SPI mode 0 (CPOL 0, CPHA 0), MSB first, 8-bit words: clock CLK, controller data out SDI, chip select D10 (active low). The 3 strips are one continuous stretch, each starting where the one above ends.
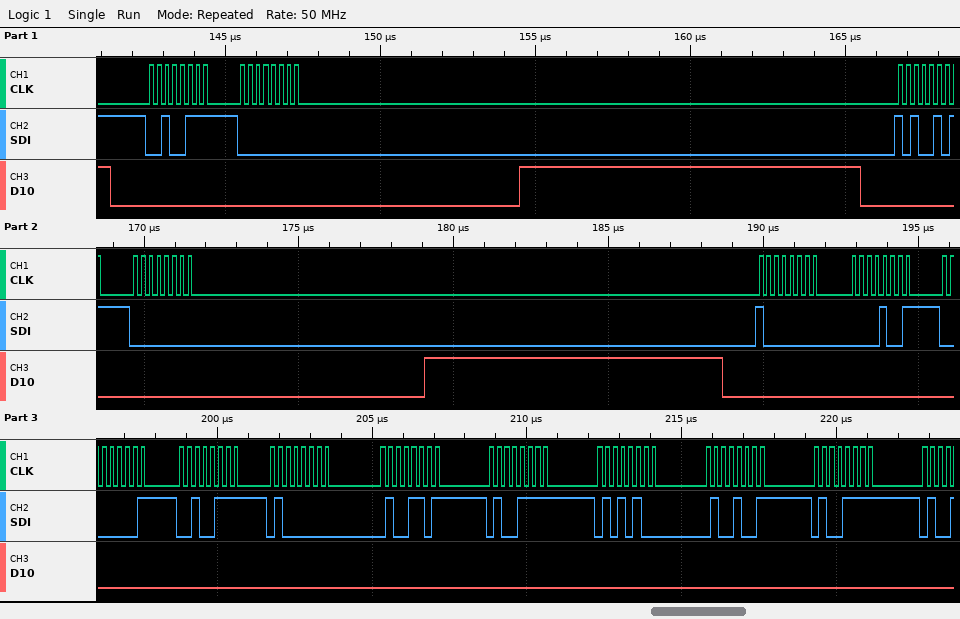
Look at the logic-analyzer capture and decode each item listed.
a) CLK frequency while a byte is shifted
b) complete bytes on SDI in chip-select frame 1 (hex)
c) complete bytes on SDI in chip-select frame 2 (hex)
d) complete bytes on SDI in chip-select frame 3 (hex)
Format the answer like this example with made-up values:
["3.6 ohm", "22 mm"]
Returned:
["4 MHz", "27 00", "A5 00", "80 09 01 27 40 4D 4F 54 49 4F"]
